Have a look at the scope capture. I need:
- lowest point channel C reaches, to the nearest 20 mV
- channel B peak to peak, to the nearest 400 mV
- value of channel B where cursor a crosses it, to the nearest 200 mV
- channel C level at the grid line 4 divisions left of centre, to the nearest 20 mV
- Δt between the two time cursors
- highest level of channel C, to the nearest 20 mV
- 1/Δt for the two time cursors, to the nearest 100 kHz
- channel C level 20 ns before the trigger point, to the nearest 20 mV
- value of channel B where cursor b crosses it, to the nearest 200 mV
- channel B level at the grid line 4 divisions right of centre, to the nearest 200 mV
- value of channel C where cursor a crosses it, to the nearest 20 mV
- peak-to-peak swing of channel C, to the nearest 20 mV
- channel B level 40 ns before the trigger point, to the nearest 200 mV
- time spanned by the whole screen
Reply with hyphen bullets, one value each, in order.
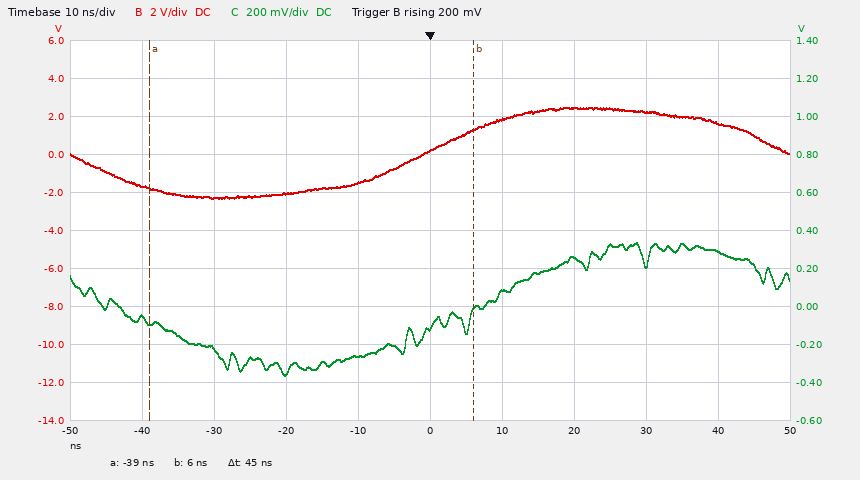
- -360 mV
- 4.8 V
- -1.8 V
- -60 mV
- 45 ns
- 340 mV
- 22.2 MHz
- -340 mV
- 1.2 V
- 1.6 V
- -80 mV
- 700 mV
- -1.6 V
- 100 ns
